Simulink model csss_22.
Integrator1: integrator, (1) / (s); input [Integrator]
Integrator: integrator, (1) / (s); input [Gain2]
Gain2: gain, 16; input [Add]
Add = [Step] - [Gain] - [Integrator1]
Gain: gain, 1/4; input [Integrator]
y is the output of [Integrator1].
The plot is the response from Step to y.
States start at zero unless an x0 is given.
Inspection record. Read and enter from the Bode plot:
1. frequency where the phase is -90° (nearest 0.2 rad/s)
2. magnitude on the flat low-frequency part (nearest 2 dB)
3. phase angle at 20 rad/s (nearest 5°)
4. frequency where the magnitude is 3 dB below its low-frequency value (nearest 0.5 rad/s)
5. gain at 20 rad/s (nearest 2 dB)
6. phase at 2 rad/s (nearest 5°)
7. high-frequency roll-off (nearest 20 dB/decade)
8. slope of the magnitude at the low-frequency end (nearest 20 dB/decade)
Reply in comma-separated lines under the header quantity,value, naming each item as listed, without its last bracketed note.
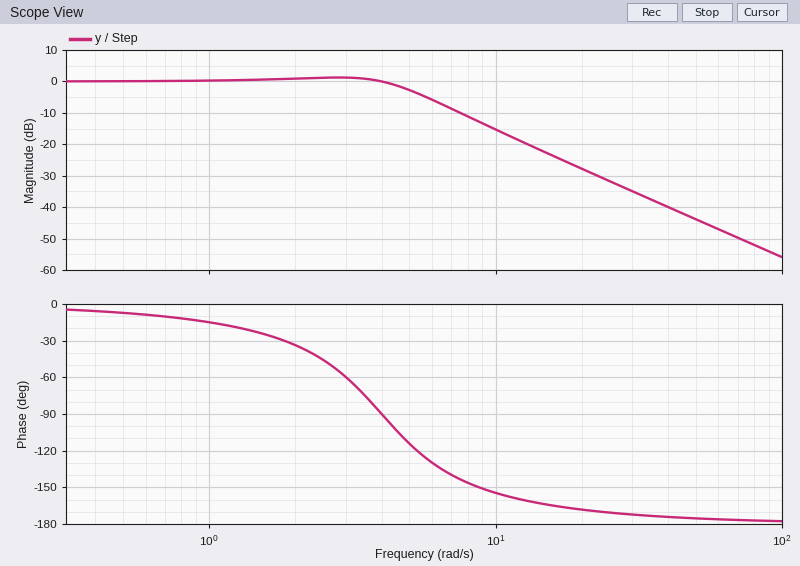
quantity,value
frequency where the phase is -90°,4.0 rad/s
magnitude on the flat low-frequency part,0 dB
phase angle at 20 rad/s,-170°
frequency where the magnitude is 3 dB below its low-frequency value,5.0 rad/s
gain at 20 rad/s,-28 dB
phase at 2 rad/s,-35°
high-frequency roll-off,-40 dB/decade
slope of the magnitude at the low-frequency end,0 dB/decade
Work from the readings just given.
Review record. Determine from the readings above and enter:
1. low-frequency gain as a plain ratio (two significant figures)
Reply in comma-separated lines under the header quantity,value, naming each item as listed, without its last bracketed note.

quantity,value
low-frequency gain as a plain ratio,1.0
